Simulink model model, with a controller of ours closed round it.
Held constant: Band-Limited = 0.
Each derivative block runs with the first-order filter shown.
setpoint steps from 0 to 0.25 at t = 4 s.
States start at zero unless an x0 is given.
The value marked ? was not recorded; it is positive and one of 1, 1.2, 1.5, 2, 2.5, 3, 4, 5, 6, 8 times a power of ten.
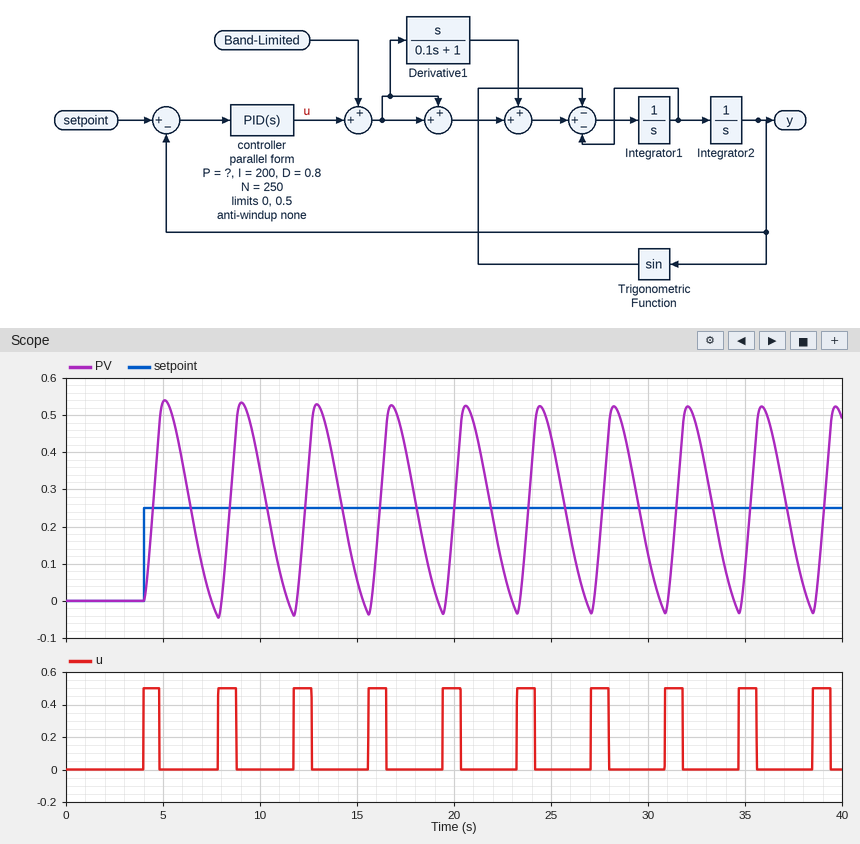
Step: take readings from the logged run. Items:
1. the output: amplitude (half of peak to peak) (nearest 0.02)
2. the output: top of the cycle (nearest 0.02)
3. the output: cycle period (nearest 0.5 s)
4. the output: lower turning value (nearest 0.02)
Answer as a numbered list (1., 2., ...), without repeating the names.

1. 0.28
2. 0.52
3. 4.0 s
4. -0.04
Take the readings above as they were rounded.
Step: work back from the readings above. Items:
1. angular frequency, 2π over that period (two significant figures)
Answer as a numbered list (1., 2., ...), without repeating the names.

1. 1.6 rad/s
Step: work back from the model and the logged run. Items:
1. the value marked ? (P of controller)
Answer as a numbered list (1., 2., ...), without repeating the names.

1. 25
